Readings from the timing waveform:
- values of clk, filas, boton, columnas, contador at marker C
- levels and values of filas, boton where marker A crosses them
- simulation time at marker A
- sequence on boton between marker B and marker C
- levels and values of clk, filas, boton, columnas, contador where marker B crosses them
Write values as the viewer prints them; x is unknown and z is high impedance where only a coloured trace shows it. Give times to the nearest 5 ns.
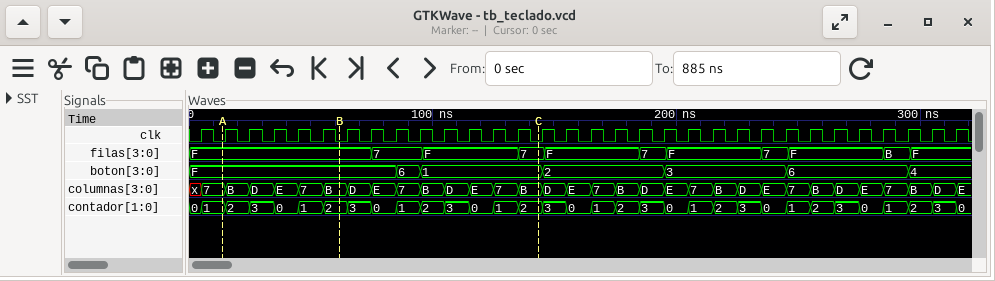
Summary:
clk=0, filas=7, boton=1, columnas=B, contador=2
filas=F, boton=F
15 ns
F, 6, 1
clk=0, filas=F, boton=F, columnas=B, contador=2
